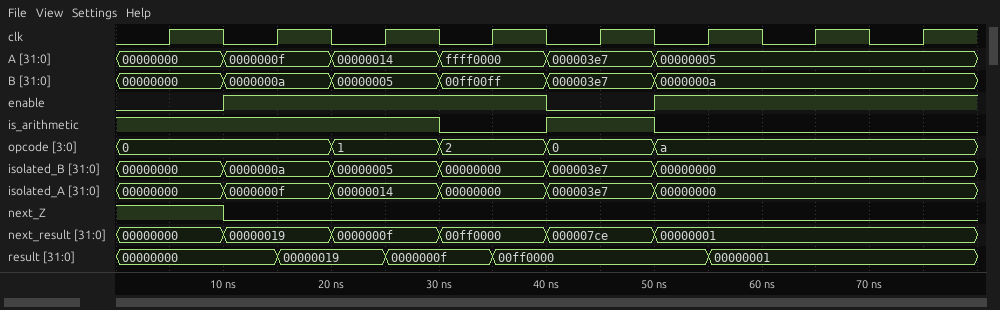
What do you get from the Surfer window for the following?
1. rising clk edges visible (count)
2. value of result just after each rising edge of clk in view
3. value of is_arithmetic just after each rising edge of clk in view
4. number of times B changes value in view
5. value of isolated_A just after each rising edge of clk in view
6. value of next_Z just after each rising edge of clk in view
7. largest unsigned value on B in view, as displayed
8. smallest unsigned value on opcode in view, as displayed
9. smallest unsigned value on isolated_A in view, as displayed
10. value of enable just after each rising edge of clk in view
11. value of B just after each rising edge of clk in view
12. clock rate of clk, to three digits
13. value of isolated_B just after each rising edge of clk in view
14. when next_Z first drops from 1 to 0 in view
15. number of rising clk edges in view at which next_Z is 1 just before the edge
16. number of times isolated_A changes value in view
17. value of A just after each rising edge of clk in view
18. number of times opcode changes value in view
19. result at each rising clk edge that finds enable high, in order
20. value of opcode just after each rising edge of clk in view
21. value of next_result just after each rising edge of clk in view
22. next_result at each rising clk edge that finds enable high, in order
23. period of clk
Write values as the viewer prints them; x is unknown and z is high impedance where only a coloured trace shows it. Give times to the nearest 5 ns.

8
00000000, 00000019, 0000000f, 00ff0000, 00ff0000, 00000001, 00000001, 00000001
1 1 1 0 1 0 0 0
5
00000000, 0000000f, 00000014, 00000000, 000003e7, 00000000, 00000000, 00000000
1 0 0 0 0 0 0 0
00ff00ff
0
00000000
0 1 1 1 0 1 1 1
00000000, 0000000a, 00000005, 00ff00ff, 000003e7, 0000000a, 0000000a, 0000000a
100 MHz
00000000, 0000000a, 00000005, 00000000, 000003e7, 00000000, 00000000, 00000000
10 ns
1
5
00000000, 0000000f, 00000014, ffff0000, 000003e7, 00000005, 00000005, 00000005
4
00000000, 00000019, 0000000f, 00ff0000, 00000001, 00000001
0, 0, 1, 2, 0, a, a, a
00000000, 00000019, 0000000f, 00ff0000, 000007ce, 00000001, 00000001, 00000001
00000019, 0000000f, 00ff0000, 00000001, 00000001, 00000001
10 ns
